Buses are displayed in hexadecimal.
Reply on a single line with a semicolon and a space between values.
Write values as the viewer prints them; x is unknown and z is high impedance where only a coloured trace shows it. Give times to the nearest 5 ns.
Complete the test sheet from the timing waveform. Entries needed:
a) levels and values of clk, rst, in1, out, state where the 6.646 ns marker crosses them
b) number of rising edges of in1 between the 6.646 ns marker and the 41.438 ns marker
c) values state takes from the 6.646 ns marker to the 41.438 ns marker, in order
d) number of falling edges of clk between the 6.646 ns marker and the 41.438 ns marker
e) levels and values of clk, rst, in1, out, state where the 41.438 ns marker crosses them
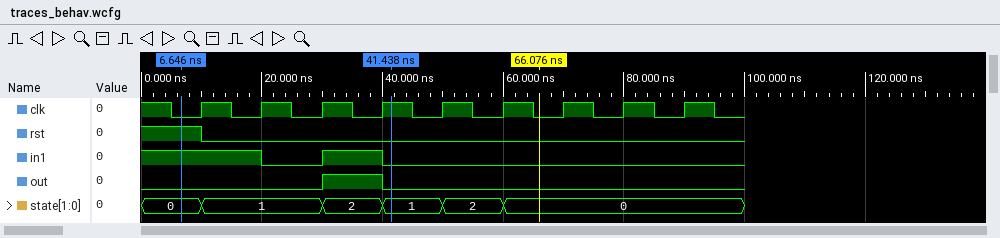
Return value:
clk=0, rst=1, in1=1, out=0, state=0; 1; 0, 1, 2, 1; 3; clk=1, rst=0, in1=0, out=0, state=1
